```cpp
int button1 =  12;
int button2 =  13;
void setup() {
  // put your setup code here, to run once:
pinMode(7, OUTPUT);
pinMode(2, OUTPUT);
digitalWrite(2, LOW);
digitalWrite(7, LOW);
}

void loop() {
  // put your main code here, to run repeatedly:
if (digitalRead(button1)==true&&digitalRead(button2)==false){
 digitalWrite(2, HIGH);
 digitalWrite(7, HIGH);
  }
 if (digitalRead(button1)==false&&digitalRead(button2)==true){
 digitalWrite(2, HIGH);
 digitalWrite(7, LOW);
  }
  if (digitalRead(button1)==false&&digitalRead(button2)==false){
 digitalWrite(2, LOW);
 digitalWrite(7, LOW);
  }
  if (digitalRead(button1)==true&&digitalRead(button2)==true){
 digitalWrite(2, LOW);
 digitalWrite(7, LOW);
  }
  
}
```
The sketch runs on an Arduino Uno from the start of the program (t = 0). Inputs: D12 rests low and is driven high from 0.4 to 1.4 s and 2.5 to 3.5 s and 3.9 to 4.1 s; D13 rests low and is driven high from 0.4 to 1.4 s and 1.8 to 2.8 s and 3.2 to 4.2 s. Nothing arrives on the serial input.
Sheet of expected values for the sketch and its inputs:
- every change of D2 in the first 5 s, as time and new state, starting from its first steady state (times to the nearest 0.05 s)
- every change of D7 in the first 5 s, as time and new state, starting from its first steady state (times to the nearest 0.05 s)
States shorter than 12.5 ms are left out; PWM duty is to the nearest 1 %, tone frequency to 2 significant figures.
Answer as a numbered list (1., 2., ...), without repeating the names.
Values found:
1. 0 s low; 1.8 s high; 2.5 s low; 2.8 s high; 3.2 s low; 3.5 s high; 3.9 s low; 4.1 s high; 4.2 s low
2. 0 s low; 2.8 s high; 3.2 s low
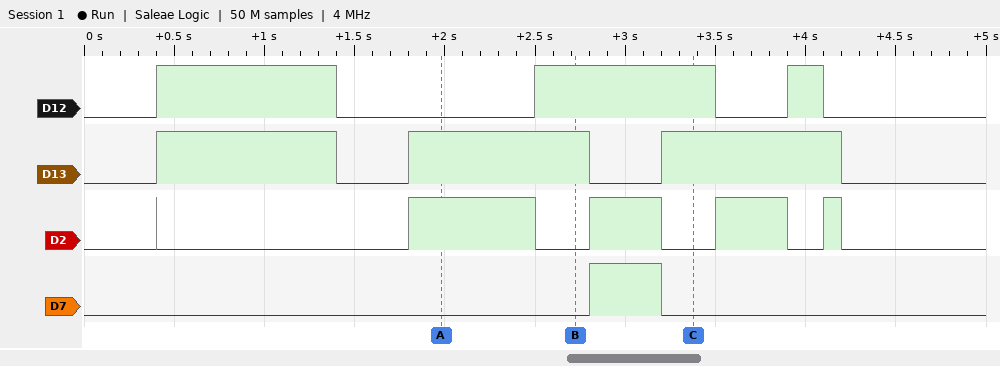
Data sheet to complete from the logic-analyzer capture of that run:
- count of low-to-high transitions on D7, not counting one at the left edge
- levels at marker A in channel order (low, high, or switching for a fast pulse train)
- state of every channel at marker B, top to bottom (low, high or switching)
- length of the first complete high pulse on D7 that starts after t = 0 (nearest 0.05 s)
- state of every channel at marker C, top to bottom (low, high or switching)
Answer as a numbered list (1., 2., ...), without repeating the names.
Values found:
1. 1
2. D12 low, D13 high, D2 high, D7 low
3. D12 high, D13 high, D2 low, D7 low
4. 0.40 s
5. D12 high, D13 high, D2 low, D7 low
